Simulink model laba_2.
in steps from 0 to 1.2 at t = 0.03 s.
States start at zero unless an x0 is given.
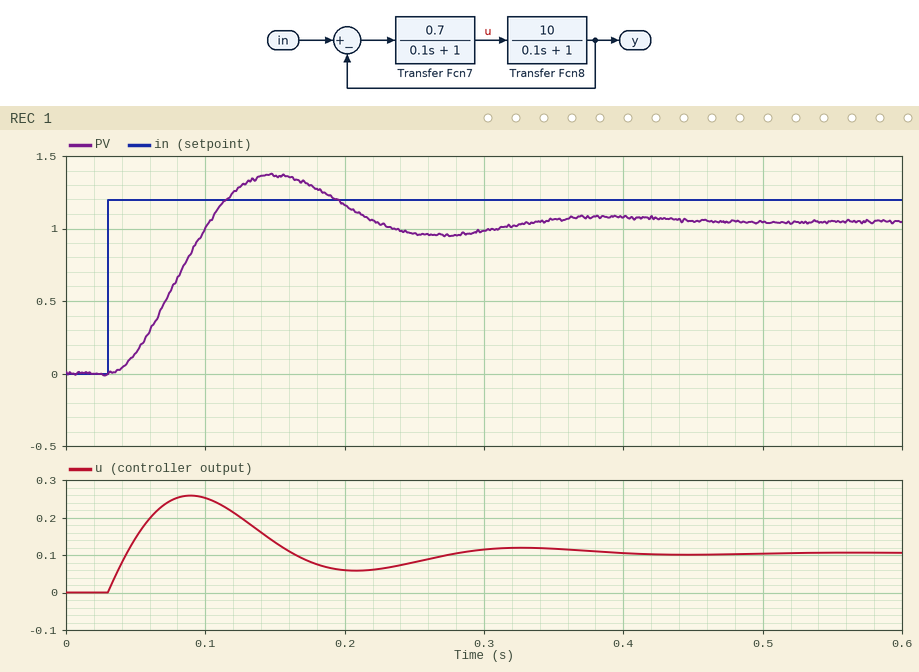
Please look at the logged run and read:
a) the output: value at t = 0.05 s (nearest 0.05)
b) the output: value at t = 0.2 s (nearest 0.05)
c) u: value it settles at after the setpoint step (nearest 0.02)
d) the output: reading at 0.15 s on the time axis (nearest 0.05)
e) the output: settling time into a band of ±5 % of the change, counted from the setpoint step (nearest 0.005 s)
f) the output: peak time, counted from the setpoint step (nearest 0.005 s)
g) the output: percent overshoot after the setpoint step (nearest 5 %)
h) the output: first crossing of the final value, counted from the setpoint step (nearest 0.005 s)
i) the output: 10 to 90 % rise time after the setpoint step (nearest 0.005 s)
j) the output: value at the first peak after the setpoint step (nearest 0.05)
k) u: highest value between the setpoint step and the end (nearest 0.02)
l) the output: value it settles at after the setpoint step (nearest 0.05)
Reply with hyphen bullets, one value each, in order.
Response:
- 0.15
- 1.15
- 0.10
- 1.35
- 0.280 s
- 0.120 s
- 30 %
- 0.075 s
- 0.050 s
- 1.35
- 0.26
- 1.05
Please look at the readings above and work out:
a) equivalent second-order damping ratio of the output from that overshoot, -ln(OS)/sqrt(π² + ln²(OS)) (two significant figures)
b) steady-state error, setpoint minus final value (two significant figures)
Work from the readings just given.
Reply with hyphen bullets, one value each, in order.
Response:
- 0.36
- 0.15
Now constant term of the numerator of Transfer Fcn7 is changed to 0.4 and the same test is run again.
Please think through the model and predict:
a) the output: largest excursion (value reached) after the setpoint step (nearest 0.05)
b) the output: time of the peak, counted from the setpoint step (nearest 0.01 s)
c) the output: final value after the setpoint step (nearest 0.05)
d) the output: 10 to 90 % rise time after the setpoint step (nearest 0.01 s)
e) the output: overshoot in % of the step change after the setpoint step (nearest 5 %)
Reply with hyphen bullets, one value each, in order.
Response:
- 1.15
- 0.16 s
- 0.95
- 0.07 s
- 20 %
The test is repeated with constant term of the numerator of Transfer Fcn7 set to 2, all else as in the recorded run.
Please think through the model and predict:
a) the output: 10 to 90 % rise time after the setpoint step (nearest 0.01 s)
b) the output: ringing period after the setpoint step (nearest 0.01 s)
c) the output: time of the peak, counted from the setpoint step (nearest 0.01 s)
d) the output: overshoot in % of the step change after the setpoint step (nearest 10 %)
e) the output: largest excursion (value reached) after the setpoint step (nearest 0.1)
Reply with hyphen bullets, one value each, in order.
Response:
- 0.03 s
- 0.14 s
- 0.07 s
- 50 %
- 1.7
